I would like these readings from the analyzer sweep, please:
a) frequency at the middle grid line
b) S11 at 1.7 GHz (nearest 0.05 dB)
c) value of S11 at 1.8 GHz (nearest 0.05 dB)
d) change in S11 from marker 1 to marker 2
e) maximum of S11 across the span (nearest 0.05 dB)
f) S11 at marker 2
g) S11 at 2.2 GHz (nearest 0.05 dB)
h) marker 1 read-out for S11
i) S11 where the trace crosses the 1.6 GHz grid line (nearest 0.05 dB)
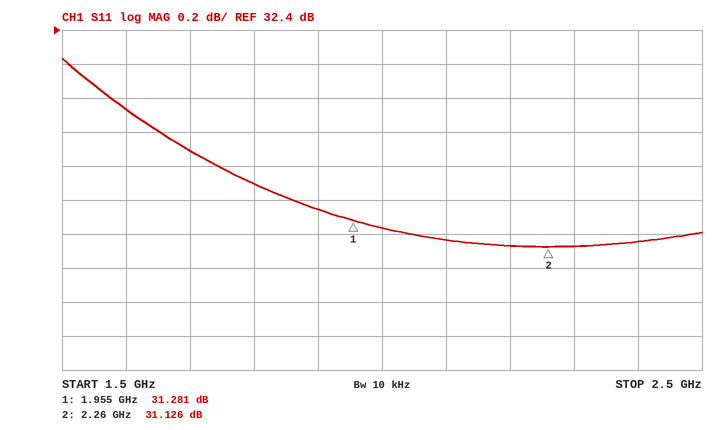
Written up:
2 GHz
31.70 dB
31.50 dB
-0.155 dB
32.25 dB
31.126 dB
31.15 dB
31.281 dB
31.95 dB
